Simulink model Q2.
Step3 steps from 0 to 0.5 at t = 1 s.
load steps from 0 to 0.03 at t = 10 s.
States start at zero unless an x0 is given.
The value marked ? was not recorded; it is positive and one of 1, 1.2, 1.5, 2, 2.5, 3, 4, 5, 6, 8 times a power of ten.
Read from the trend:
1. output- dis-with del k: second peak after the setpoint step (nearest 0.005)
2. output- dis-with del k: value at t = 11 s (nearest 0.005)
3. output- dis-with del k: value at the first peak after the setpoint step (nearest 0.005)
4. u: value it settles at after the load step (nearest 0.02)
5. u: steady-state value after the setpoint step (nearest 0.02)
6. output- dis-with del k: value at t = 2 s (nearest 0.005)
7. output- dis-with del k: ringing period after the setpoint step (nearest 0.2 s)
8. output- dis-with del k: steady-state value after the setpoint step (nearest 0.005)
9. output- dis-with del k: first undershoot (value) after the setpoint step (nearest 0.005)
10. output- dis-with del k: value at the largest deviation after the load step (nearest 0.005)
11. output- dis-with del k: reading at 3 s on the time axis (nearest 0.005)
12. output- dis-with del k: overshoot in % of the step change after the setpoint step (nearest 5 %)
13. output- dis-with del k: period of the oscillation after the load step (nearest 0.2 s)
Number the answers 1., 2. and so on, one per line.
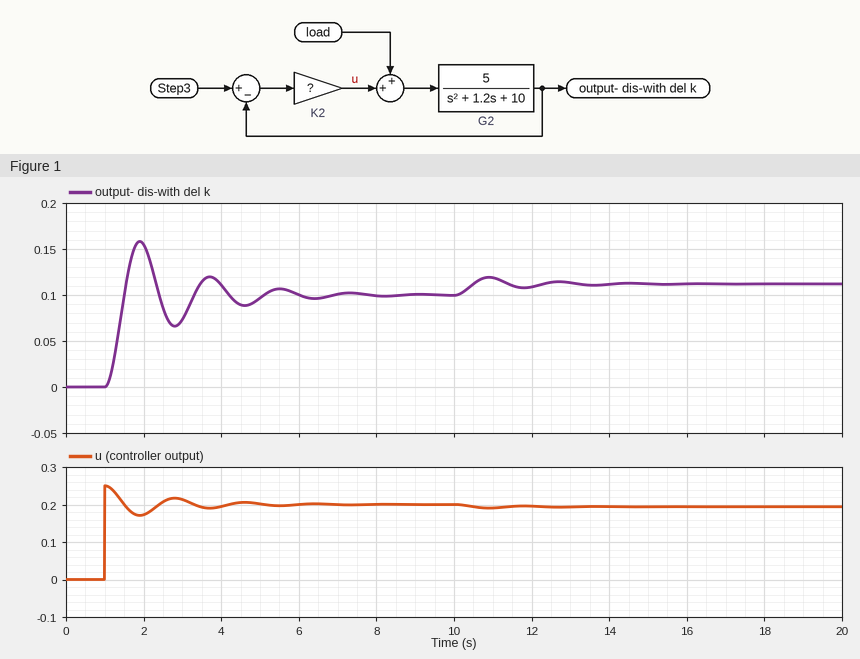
1. 0.120
2. 0.120
3. 0.160
4. 0.20
5. 0.20
6. 0.155
7. 1.8 s
8. 0.100
9. 0.065
10. 0.120
11. 0.075
12. 60 %
13. 1.8 s
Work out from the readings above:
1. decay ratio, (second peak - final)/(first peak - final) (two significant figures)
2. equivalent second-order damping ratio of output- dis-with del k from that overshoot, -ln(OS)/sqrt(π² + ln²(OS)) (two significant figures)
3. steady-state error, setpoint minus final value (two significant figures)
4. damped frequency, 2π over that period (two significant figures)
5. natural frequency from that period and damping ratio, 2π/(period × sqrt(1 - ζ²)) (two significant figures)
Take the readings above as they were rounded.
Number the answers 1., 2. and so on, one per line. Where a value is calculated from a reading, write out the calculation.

1. (0.12 - 0.1) / (0.16 - 0.1) = 0.33
2. ln(0.6) = -0.511; 0.511 / sqrt(9.870 + 0.261) = 0.16
3. 0.5 - 0.1 = 0.40
4. 2π / 1.8 = 3.5 rad/s
5. 2π / (1.8 × sqrt(1 - 0.16²)) = 3.5 rad/s
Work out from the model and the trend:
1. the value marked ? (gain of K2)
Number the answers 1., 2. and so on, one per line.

1. 0.5
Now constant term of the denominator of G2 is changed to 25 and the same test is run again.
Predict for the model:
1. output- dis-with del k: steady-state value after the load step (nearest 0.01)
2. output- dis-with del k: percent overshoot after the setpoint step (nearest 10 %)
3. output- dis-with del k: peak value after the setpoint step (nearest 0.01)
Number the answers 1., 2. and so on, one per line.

1. 0.05
2. 70 %
3. 0.08
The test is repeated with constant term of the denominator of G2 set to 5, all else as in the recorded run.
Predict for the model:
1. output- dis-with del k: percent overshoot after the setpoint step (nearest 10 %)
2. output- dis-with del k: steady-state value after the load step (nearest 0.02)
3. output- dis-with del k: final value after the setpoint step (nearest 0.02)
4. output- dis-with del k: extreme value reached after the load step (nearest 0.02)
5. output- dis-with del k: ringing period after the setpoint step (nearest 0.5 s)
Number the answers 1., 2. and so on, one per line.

1. 50 %
2. 0.18
3. 0.16
4. 0.20
5. 2.5 s
